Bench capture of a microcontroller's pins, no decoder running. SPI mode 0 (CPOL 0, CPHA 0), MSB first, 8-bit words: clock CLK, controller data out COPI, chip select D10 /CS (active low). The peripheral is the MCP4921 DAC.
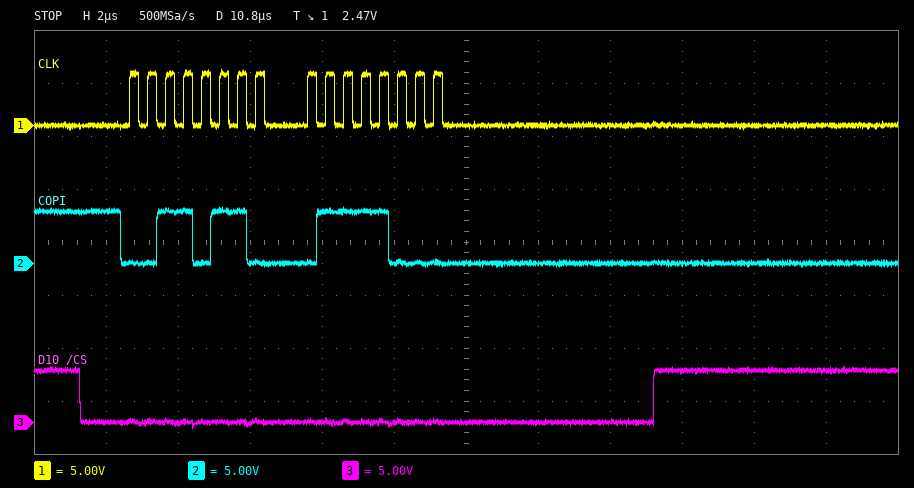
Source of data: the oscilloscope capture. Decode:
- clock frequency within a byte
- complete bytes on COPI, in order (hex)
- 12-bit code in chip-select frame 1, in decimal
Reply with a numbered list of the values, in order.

1. 2 MHz
2. 36 78
3. 1656
